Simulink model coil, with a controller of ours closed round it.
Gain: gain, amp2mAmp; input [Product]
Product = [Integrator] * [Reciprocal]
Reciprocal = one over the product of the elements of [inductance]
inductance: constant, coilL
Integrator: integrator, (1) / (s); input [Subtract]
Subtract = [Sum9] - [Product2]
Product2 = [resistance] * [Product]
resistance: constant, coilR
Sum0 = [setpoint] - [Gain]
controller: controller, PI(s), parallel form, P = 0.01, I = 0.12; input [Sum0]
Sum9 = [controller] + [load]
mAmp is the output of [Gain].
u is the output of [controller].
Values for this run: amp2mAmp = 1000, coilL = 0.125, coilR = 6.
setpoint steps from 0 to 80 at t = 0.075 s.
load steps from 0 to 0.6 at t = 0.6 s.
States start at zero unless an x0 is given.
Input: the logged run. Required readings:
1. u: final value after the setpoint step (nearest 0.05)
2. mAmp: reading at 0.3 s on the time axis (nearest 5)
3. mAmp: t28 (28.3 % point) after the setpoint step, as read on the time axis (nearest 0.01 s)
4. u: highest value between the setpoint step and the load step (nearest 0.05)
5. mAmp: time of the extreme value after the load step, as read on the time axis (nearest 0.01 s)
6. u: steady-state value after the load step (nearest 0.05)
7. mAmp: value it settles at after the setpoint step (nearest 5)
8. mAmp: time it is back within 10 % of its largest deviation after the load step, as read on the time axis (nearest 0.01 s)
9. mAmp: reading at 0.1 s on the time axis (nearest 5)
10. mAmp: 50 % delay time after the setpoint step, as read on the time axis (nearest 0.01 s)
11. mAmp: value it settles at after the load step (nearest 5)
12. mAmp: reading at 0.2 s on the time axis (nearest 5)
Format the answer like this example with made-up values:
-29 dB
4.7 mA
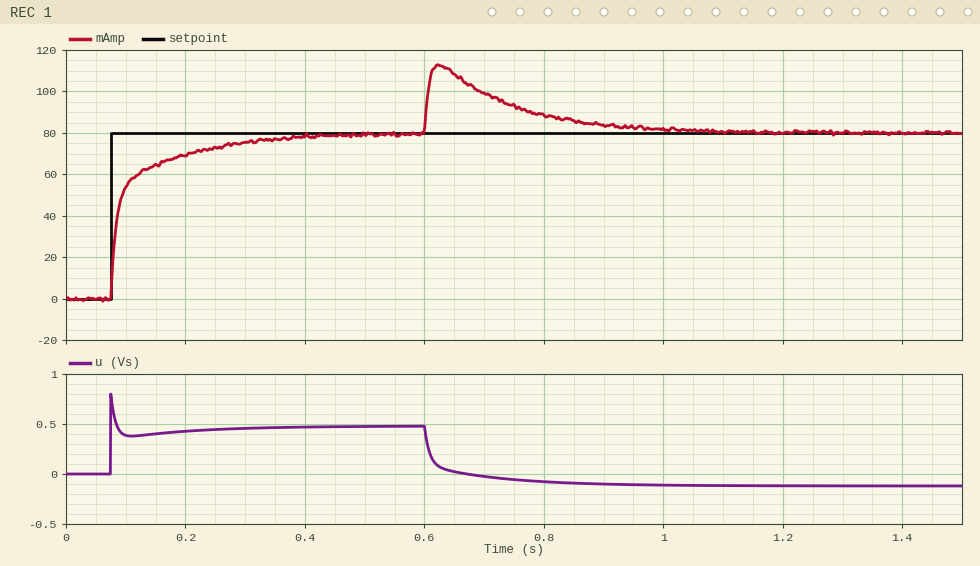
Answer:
0.50
75
0.08 s
0.80
0.62 s
-0.10
80
0.92 s
55
0.09 s
80
70
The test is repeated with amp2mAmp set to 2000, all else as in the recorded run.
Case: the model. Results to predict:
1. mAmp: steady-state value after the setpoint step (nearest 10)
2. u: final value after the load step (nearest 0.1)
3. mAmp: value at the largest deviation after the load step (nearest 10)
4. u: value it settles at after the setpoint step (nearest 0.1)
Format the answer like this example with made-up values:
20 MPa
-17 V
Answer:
80
-0.4
120
0.2
